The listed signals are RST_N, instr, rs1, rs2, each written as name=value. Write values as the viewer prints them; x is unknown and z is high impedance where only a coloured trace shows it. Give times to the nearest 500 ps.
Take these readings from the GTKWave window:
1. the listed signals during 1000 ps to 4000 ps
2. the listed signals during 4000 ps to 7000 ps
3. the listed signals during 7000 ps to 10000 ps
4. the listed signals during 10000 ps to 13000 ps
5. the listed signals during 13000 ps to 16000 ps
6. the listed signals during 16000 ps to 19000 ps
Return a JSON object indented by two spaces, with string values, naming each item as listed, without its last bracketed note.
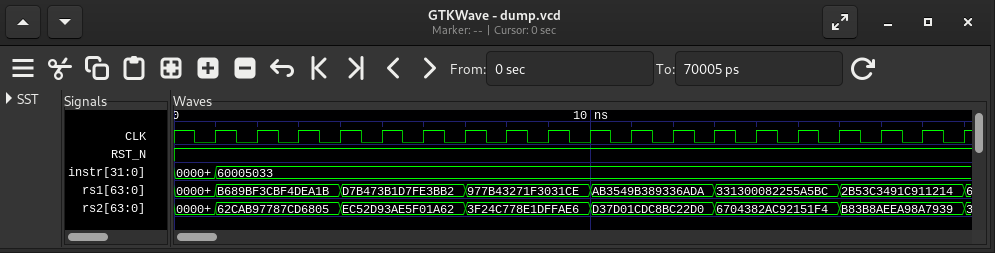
{
  "the listed signals during 1000 ps to 4000 ps": "RST_N=1, instr=60005033, rs1=B689BF3CBF4DEA1B, rs2=62CAB97787CD6805",
  "the listed signals during 4000 ps to 7000 ps": "RST_N=1, instr=60005033, rs1=D7B473B1D7FE3BB2, rs2=EC52D93AE5F01A62",
  "the listed signals during 7000 ps to 10000 ps": "RST_N=1, instr=60005033, rs1=977B43271F3031CE, rs2=3F24C778E1DFFAE6",
  "the listed signals during 10000 ps to 13000 ps": "RST_N=1, instr=60005033, rs1=AB3549B389336ADA, rs2=D37D01CDC8BC22D0",
  "the listed signals during 13000 ps to 16000 ps": "RST_N=1, instr=60005033, rs1=331300082255A5BC, rs2=6704382AC92151F4",
  "the listed signals during 16000 ps to 19000 ps": "RST_N=1, instr=60005033, rs1=2B53C3491C911214, rs2=B83B8AEEA98A7939"
}
